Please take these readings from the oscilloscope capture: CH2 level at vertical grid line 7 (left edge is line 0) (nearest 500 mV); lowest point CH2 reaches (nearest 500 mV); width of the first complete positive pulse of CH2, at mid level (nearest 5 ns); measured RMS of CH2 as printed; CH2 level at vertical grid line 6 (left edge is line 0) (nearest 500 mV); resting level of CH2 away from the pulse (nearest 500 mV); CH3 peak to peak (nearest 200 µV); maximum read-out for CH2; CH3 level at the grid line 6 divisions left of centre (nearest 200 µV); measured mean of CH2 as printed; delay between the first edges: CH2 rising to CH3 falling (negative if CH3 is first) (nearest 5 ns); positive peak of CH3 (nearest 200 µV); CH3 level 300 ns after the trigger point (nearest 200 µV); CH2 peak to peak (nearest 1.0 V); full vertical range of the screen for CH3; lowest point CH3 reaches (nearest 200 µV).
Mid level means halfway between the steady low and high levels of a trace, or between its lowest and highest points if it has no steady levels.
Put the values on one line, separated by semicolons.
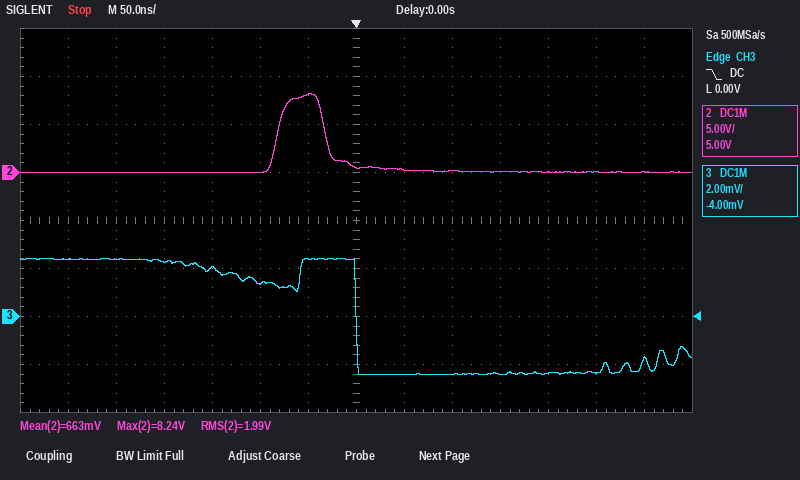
500 mV; 0.0 V; 50 ns; 1.99 V; 8.0 V; 0.0 V; 4.8 mV; 8.24 V; 2.4 mV; 663 mV; +80 ns; 2.4 mV; -1.8 mV; 8.0 V; 16 mV; -2.4 mV
